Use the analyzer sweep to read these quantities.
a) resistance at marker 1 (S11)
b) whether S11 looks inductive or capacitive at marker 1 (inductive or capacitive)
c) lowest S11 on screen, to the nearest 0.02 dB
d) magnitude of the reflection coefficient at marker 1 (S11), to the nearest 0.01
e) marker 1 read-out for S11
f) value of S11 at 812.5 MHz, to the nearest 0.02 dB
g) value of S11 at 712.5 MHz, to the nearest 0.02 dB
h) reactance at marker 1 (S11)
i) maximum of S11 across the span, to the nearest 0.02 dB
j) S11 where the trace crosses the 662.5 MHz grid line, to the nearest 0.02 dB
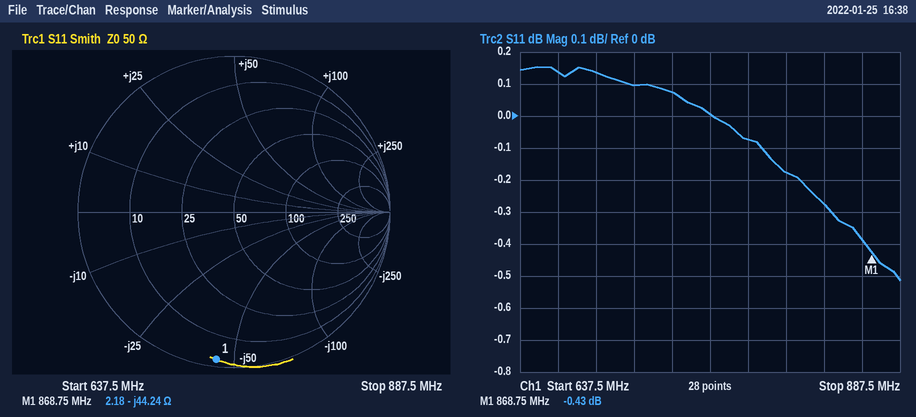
2.18 Ω
capacitive
-0.52 dB
0.95
-0.43 dB
-0.18 dB
0.10 dB
-44.24 Ω
0.16 dB
0.14 dB
